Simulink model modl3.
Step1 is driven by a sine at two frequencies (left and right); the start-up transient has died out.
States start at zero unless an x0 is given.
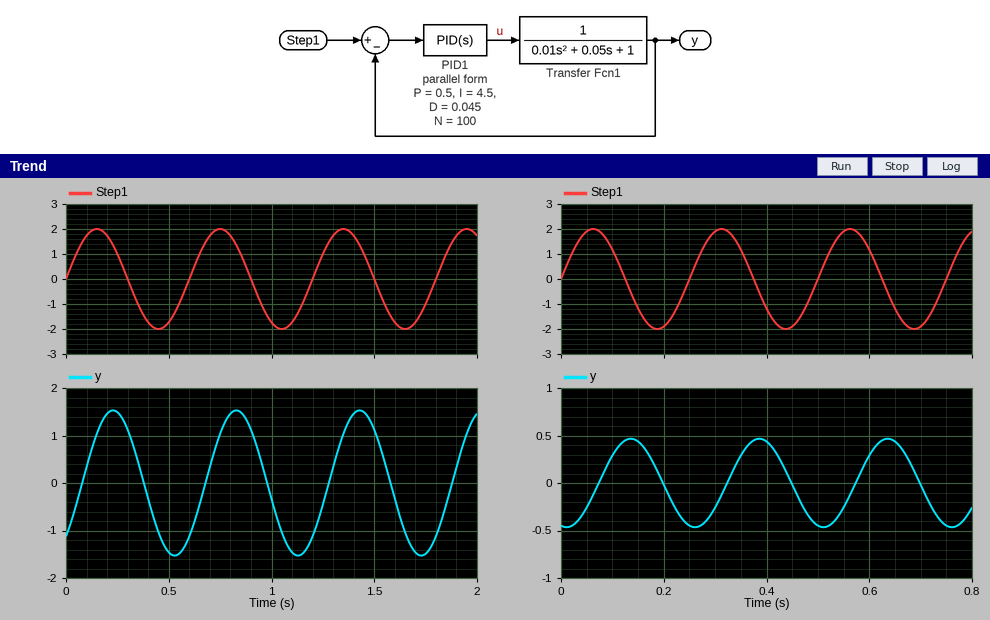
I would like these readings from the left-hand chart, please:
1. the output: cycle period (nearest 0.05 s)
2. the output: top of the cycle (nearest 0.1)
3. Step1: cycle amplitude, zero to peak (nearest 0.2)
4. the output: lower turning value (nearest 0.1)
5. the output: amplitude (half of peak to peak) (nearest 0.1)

0.60 s
1.5
2.0
-1.5
1.5
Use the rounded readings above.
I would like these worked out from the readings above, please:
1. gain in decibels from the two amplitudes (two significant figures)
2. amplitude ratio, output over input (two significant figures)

-2.5 dB
0.75
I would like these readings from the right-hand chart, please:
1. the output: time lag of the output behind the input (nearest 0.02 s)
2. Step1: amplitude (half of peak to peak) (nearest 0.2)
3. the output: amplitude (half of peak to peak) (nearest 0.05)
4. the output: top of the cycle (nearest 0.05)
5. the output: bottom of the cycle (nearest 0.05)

0.08 s
2.0
0.45
0.45
-0.45
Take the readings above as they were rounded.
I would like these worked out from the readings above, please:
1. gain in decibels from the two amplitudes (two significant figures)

-13 dB
